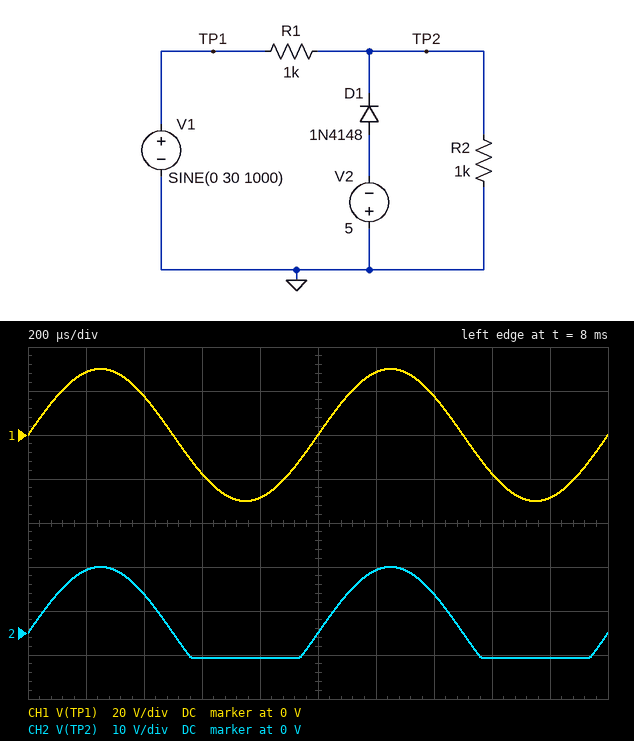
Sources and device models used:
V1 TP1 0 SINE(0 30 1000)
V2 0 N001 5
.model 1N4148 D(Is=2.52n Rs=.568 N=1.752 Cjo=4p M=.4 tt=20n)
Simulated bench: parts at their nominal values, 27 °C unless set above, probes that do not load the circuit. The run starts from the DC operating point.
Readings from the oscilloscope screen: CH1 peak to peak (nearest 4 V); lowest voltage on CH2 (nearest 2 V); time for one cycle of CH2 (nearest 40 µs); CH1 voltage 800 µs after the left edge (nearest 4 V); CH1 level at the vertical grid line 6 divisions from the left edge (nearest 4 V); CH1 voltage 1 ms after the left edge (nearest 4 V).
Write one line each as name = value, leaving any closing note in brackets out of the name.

CH1 peak to peak = 60 V
lowest voltage on CH2 = -6 V
time for one cycle of CH2 = 1.00 ms
CH1 voltage 800 µs after the left edge = -28 V
CH1 level at the vertical grid line 6 divisions from the left edge = 28 V
CH1 voltage 1 ms after the left edge = 0 V
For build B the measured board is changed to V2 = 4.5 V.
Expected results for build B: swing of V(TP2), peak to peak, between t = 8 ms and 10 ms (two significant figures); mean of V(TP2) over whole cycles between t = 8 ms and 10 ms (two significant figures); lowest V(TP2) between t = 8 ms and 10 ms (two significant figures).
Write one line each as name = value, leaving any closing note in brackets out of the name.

swing of V(TP2), peak to peak, between t = 8 ms and 10 ms = 20 V
mean of V(TP2) over whole cycles between t = 8 ms and 10 ms = 2.5 V
lowest V(TP2) between t = 8 ms and 10 ms = -5.2 V
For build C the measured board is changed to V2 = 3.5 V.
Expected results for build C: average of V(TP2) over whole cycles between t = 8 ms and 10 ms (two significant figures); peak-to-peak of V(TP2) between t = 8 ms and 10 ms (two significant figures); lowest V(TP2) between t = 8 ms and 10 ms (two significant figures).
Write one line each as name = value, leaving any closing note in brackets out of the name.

average of V(TP2) over whole cycles between t = 8 ms and 10 ms = 2.9 V
peak-to-peak of V(TP2) between t = 8 ms and 10 ms = 19 V
lowest V(TP2) between t = 8 ms and 10 ms = -4.2 V
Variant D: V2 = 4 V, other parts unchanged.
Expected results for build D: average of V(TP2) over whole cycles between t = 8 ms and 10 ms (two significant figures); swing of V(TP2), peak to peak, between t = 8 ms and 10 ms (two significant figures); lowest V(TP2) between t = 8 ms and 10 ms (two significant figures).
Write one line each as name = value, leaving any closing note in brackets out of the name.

average of V(TP2) over whole cycles between t = 8 ms and 10 ms = 2.7 V
swing of V(TP2), peak to peak, between t = 8 ms and 10 ms = 20 V
lowest V(TP2) between t = 8 ms and 10 ms = -4.7 V
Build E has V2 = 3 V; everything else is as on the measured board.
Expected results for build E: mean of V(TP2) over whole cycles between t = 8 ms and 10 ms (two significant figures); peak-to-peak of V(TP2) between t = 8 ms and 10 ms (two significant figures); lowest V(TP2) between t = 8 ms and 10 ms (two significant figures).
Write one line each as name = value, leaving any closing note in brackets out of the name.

mean of V(TP2) over whole cycles between t = 8 ms and 10 ms = 3.1 V
peak-to-peak of V(TP2) between t = 8 ms and 10 ms = 19 V
lowest V(TP2) between t = 8 ms and 10 ms = -3.7 V
